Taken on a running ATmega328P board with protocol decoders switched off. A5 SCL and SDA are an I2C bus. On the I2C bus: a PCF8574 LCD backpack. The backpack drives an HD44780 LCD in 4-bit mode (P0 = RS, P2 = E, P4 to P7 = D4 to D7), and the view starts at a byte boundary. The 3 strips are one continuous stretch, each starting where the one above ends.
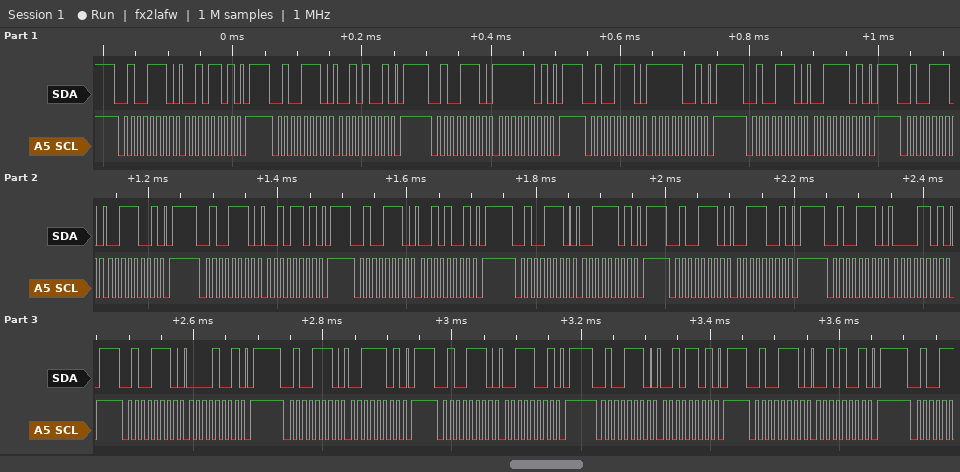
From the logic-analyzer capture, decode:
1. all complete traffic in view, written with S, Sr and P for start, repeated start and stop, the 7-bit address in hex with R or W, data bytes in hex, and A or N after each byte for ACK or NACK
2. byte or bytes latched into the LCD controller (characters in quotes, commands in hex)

S 27W A 2D A P S 27W A 29 A P S 27W A FD A P S 27W A F9 A P S 27W A 3D A P S 27W A 39 A P S 27W A 2D A P S 27W A 29 A P S 27W A 3D A P S 27W A 39 A P S 27W A 0D A P S 27W A 09 A P S 27W A 3D A P S 27W A 39 A P S 27W A 2D A P S 27W A 29 A P
'/' '2' '0' '2'
